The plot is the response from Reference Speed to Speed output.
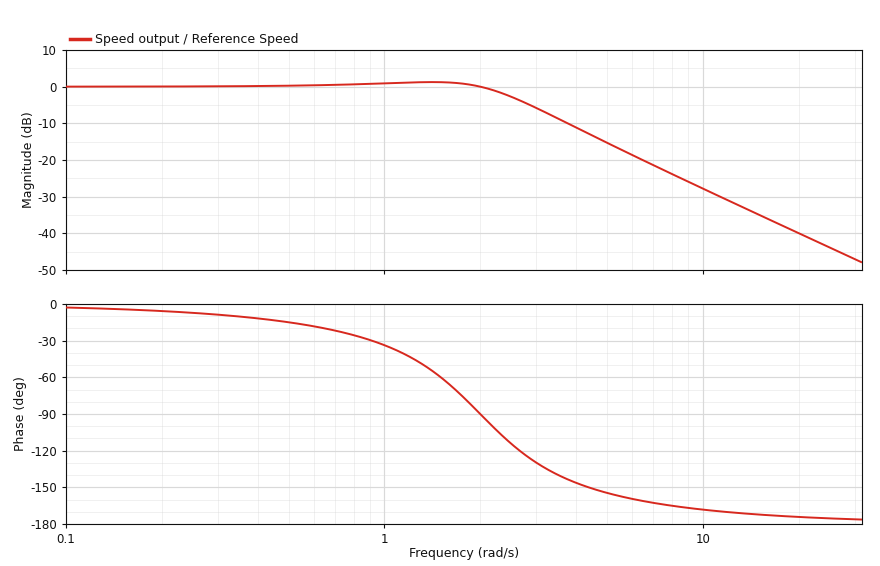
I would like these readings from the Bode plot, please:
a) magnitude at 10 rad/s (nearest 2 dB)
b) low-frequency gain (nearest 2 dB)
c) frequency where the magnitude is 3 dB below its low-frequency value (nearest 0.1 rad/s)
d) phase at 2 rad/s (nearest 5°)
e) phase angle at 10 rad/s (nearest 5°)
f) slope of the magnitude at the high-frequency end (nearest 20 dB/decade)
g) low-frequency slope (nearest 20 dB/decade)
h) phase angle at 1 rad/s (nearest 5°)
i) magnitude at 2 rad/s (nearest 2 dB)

-28 dB
0 dB
2.5 rad/s
-90°
-170°
-40 dB/decade
0 dB/decade
-35°
0 dB
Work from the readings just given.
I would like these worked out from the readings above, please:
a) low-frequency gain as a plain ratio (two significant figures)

1.0
